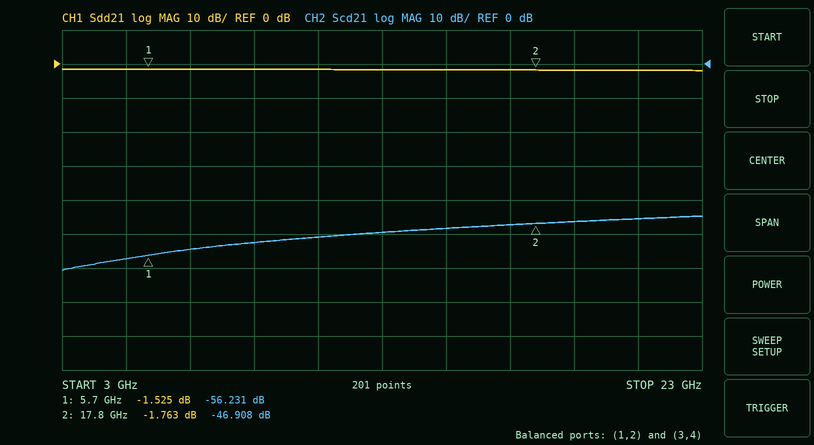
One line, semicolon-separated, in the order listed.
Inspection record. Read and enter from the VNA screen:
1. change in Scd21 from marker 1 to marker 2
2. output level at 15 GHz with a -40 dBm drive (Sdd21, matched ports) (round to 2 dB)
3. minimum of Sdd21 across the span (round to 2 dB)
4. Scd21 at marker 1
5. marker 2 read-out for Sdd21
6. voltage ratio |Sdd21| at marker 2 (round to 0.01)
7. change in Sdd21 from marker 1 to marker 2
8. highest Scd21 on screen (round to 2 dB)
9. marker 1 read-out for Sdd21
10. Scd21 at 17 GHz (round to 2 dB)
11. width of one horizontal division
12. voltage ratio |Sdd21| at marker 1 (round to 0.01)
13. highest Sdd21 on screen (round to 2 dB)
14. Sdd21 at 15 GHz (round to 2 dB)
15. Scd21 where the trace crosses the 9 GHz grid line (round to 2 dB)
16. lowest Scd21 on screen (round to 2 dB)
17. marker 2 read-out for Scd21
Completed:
9.323 dB; -42 dBm; -2 dB; -56.231 dB; -1.763 dB; 0.82; -0.238 dB; -44 dB; -1.525 dB; -48 dB; 2 GHz; 0.84; -2 dB; -2 dB; -52 dB; -60 dB; -46.908 dB
